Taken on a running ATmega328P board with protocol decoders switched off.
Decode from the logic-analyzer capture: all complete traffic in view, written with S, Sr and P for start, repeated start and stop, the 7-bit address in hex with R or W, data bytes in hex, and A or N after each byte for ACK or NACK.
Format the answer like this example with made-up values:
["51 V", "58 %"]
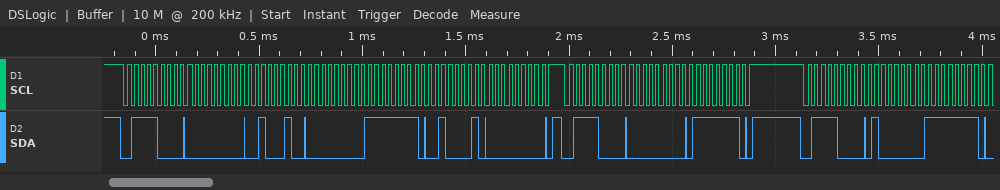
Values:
["S 3CW A 00 A 22 A 00 A FF A 21 A 00 A P S 3CW A 00 A 7F A P S 3CW A 40 A FF A"]
